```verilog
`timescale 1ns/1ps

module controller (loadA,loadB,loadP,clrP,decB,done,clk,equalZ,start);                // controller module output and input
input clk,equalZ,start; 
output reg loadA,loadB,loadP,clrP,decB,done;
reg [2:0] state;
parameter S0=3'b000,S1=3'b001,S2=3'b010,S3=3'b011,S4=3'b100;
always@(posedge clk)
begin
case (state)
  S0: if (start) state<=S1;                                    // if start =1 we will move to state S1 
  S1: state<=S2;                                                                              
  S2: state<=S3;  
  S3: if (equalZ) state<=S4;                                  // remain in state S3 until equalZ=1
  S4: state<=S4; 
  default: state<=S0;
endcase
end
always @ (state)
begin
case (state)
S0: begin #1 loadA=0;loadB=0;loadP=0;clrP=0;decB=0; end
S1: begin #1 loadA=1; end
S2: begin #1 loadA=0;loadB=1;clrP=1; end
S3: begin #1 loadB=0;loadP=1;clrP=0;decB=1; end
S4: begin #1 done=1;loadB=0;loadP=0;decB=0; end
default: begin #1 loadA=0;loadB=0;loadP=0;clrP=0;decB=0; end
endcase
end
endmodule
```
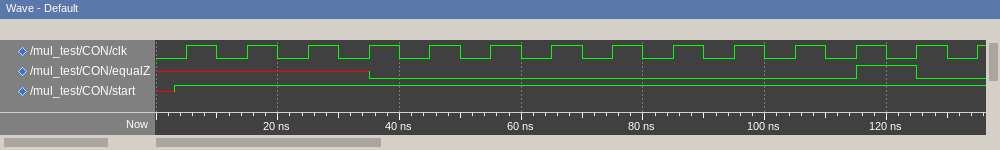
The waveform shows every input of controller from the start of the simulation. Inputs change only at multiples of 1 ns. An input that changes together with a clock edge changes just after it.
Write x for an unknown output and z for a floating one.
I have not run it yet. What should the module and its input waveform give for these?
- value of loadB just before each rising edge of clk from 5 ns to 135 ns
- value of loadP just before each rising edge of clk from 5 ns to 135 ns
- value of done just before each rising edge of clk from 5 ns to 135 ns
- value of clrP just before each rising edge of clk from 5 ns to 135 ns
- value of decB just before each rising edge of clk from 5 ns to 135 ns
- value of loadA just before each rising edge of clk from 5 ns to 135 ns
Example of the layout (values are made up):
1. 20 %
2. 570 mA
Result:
1. x 0 0 1 0 0 0 0 0 0 0 0 0 0
2. x 0 0 0 1 1 1 1 1 1 1 1 1 0
3. x x x x x x x x x x x x x 1
4. x 0 0 1 0 0 0 0 0 0 0 0 0 0
5. x 0 0 0 1 1 1 1 1 1 1 1 1 0
6. x 0 1 0 0 0 0 0 0 0 0 0 0 0
